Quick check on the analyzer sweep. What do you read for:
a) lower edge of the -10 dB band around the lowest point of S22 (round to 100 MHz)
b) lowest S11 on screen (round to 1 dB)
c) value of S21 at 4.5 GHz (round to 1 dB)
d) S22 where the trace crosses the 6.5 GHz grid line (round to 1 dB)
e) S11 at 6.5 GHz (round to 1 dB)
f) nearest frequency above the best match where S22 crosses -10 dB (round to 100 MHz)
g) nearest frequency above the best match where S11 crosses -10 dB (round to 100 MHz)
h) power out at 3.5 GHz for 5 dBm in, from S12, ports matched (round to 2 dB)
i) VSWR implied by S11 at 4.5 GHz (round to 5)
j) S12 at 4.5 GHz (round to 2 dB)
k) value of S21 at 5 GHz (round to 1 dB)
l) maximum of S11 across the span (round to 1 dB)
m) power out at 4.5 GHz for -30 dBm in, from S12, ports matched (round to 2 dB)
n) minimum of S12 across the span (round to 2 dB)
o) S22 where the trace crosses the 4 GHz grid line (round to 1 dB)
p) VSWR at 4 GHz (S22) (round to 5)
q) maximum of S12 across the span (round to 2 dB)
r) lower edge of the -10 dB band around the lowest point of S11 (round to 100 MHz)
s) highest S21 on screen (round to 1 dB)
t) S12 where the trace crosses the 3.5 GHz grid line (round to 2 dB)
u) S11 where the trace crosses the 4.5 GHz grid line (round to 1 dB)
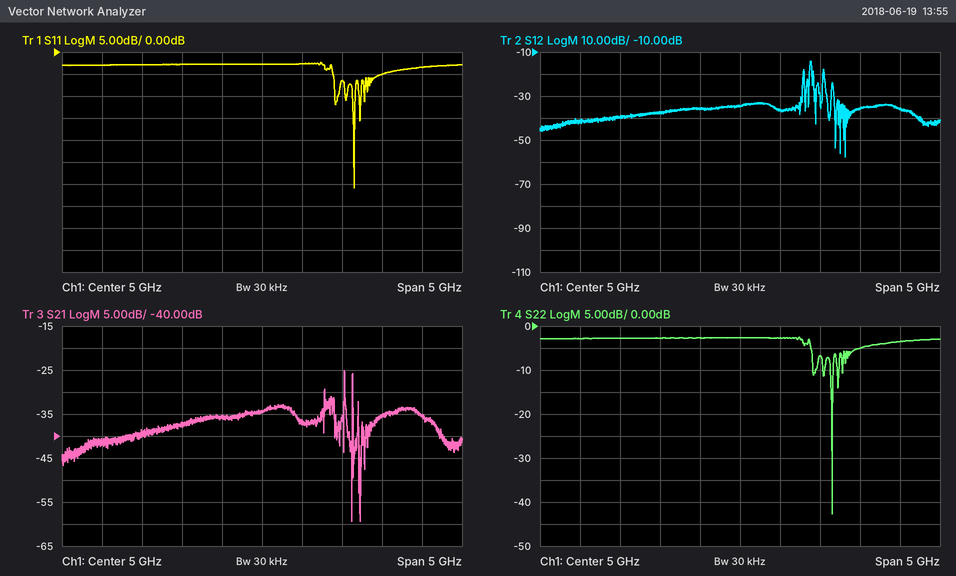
6.1 GHz
-31 dB
-36 dB
-5 dB
-5 dB
6.2 GHz
6.2 GHz
-34 dBm
5
-36 dB
-34 dB
-2 dB
-66 dBm
-58 dB
-3 dB
5
-14 dB
6.1 GHz
-25 dB
-40 dB
-3 dB
